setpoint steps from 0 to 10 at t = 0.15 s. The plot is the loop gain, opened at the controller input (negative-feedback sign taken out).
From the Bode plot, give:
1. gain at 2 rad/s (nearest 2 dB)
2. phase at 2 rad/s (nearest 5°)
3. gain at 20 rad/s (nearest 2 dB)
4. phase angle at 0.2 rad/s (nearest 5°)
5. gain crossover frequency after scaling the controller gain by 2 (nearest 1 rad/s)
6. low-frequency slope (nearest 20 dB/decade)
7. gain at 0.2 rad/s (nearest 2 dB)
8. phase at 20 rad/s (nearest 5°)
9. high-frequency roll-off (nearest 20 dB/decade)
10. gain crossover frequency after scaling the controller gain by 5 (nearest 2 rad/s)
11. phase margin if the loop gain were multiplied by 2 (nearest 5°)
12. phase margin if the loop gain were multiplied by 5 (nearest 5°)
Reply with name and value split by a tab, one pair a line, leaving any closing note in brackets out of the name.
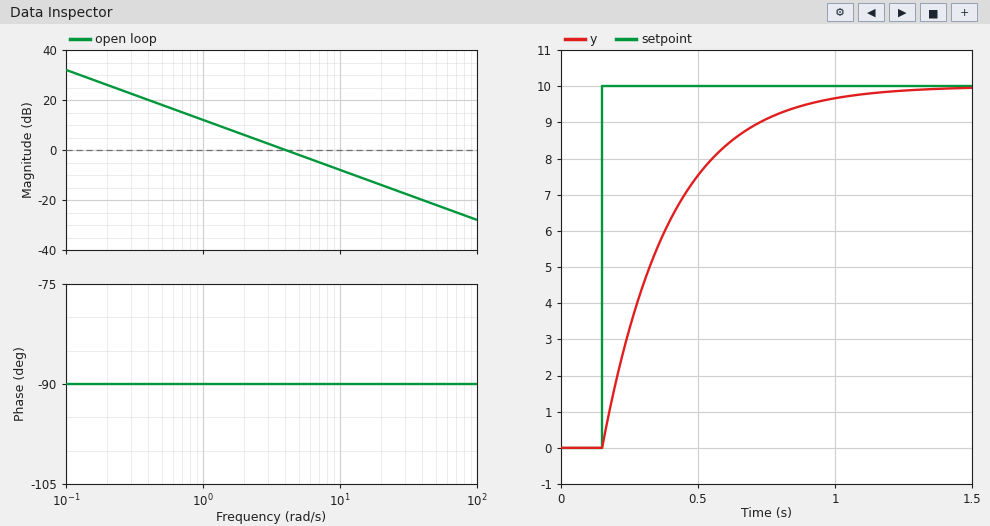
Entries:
gain at 2 rad/s	6 dB
phase at 2 rad/s	-90°
gain at 20 rad/s	-14 dB
phase angle at 0.2 rad/s	-90°
gain crossover frequency after scaling the controller gain by 2	8 rad/s
low-frequency slope	-20 dB/decade
gain at 0.2 rad/s	26 dB
phase at 20 rad/s	-90°
high-frequency roll-off	-20 dB/decade
gain crossover frequency after scaling the controller gain by 5	20 rad/s
phase margin if the loop gain were multiplied by 2	90°
phase margin if the loop gain were multiplied by 5	90°
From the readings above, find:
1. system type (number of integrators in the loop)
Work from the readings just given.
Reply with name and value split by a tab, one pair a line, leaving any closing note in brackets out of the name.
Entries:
system type	1
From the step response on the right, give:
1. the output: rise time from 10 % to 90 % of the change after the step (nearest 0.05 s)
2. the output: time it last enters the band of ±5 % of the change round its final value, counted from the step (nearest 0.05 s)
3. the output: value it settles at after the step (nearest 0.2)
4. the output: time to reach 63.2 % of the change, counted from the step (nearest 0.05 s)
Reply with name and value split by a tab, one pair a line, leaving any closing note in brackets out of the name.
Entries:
the output: rise time from 10 % to 90 % of the change after the step	0.55 s
the output: time it last enters the band of ±5 % of the change round its final value, counted from the step	0.75 s
the output: value it settles at after the step	10.0
the output: time to reach 63.2 % of the change, counted from the step	0.25 s
